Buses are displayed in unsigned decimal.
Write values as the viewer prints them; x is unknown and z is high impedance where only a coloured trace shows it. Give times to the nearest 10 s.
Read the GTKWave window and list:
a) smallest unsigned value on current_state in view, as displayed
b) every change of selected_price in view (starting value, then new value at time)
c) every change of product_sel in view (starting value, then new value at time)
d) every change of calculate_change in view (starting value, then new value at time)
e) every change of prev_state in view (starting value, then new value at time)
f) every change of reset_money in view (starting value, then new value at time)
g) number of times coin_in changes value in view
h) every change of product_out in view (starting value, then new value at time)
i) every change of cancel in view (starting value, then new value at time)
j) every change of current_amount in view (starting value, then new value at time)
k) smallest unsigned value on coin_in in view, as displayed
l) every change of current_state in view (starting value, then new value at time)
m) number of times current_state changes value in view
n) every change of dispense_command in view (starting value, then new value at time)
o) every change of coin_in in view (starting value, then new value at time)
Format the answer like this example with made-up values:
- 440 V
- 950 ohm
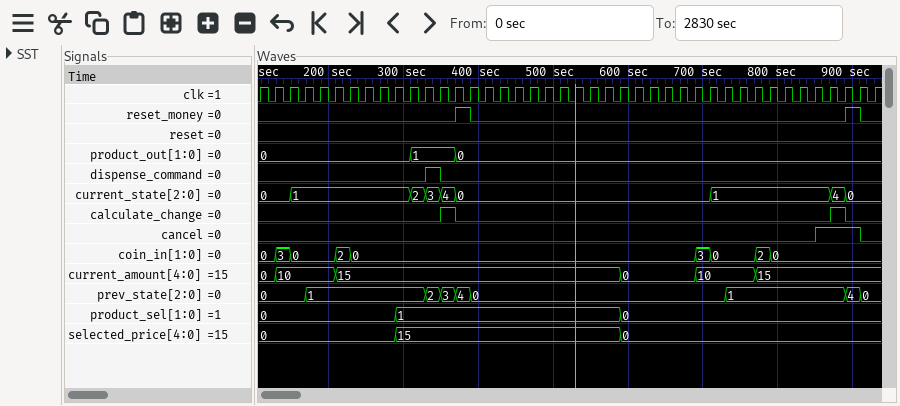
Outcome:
- 0
- 0, 15 at 290 s, 0 at 590 s
- 0, 1 at 290 s, 0 at 590 s
- 0, 1 at 350 s, 0 at 370 s, 1 at 870 s, 0 at 890 s
- 0, 1 at 170 s, 2 at 330 s, 3 at 350 s, 4 at 370 s, 0 at 390 s, 1 at 730 s, 4 at 890 s, 0 at 910 s
- 0, 1 at 370 s, 0 at 390 s, 1 at 890 s, 0 at 910 s
- 8
- 0, 1 at 310 s, 0 at 370 s
- 0, 1 at 850 s, 0 at 910 s
- 0, 10 at 130 s, 15 at 210 s, 0 at 590 s, 10 at 690 s, 15 at 770 s
- 0
- 0, 1 at 150 s, 2 at 310 s, 3 at 330 s, 4 at 350 s, 0 at 370 s, 1 at 710 s, 4 at 870 s, 0 at 890 s
- 8
- 0, 1 at 330 s, 0 at 350 s
- 0, 3 at 130 s, 0 at 150 s, 2 at 210 s, 0 at 230 s, 3 at 690 s, 0 at 710 s, 2 at 770 s, 0 at 790 s
